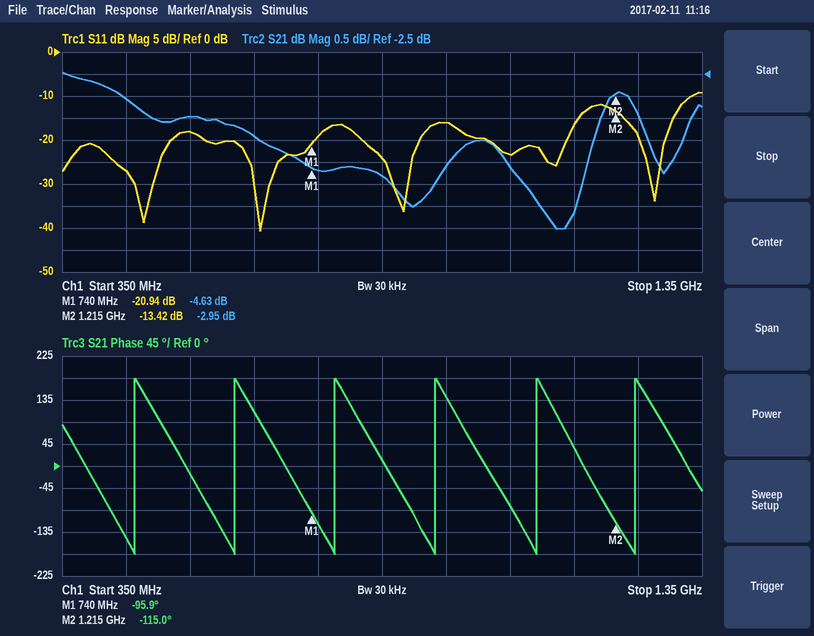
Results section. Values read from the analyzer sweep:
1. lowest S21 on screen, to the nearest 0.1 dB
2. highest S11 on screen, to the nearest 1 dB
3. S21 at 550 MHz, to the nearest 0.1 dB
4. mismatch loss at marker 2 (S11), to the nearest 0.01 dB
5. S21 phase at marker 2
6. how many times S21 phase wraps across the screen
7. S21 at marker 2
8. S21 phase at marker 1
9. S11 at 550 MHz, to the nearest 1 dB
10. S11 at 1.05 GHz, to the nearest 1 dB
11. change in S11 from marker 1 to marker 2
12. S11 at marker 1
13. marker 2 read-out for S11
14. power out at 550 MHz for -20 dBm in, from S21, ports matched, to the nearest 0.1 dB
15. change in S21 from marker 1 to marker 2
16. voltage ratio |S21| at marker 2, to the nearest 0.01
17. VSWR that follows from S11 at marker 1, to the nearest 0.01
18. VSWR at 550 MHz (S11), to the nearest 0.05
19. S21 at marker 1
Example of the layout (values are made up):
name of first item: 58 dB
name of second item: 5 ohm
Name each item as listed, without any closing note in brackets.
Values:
lowest S21 on screen, to the nearest 0.1 dB: -6.0 dB
highest S11 on screen, to the nearest 1 dB: -9 dB
S21 at 550 MHz, to the nearest 0.1 dB: -3.5 dB
mismatch loss at marker 2 (S11), to the nearest 0.01 dB: 0.20 dB
S21 phase at marker 2: -115.0°
how many times S21 phase wraps across the screen: 6
S21 at marker 2: -2.95 dB
S21 phase at marker 1: -95.9°
S11 at 550 MHz, to the nearest 1 dB: -18 dB
S11 at 1.05 GHz, to the nearest 1 dB: -23 dB
change in S11 from marker 1 to marker 2: 7.52 dB
S11 at marker 1: -20.94 dB
marker 2 read-out for S11: -13.42 dB
power out at 550 MHz for -20 dBm in, from S21, ports matched, to the nearest 0.1 dB: -23.5 dBm
change in S21 from marker 1 to marker 2: 1.68 dB
voltage ratio |S21| at marker 2, to the nearest 0.01: 0.71
VSWR that follows from S11 at marker 1, to the nearest 0.01: 1.20
VSWR at 550 MHz (S11), to the nearest 0.05: 1.30
S21 at marker 1: -4.63 dB
